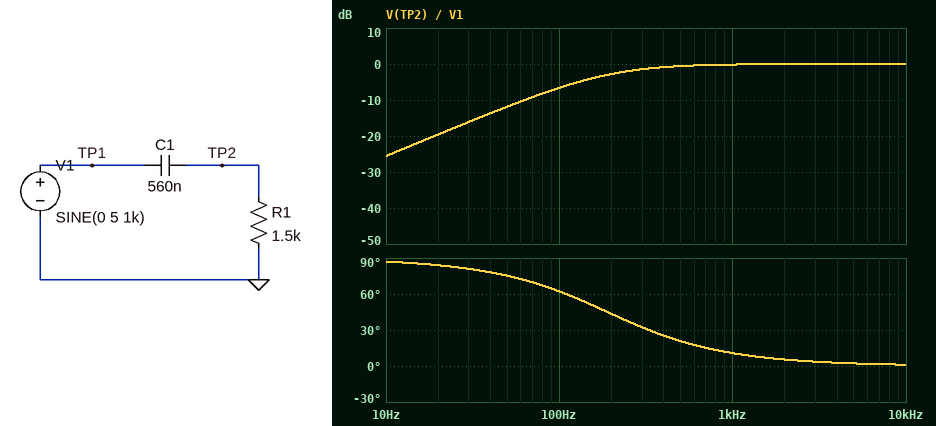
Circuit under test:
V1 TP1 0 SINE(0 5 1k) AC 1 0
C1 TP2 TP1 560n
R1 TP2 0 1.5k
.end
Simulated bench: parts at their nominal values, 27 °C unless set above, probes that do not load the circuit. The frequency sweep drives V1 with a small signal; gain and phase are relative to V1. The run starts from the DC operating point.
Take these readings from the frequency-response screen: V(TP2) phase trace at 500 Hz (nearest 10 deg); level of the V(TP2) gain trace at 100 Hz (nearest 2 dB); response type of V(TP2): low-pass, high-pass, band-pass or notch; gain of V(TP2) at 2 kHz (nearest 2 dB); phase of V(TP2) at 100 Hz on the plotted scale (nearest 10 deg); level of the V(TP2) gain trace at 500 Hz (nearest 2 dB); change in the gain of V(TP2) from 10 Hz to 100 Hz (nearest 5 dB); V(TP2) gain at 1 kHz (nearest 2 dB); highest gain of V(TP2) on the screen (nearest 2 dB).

20 deg
-6 dB
high-pass
0 dB
60 deg
0 dB
20 dB
0 dB
0 dB
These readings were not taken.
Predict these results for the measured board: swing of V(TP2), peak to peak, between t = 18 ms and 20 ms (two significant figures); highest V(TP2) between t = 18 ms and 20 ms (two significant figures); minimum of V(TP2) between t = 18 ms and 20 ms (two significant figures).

9.8 V
4.9 V
-4.9 V
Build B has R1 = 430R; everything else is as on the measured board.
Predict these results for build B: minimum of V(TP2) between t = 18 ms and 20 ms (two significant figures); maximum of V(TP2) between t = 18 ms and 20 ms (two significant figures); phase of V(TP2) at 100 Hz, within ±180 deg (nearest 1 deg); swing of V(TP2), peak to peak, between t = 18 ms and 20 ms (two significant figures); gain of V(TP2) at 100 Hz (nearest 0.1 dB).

-4.2 V
4.2 V
81 deg
8.3 V
-16.5 dB
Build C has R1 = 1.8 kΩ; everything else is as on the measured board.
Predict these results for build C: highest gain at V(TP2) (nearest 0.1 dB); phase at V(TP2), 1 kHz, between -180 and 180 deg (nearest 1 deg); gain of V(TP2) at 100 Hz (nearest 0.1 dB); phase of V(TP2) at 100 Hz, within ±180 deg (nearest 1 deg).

0 dB
9 deg
-5.4 dB
58 deg
